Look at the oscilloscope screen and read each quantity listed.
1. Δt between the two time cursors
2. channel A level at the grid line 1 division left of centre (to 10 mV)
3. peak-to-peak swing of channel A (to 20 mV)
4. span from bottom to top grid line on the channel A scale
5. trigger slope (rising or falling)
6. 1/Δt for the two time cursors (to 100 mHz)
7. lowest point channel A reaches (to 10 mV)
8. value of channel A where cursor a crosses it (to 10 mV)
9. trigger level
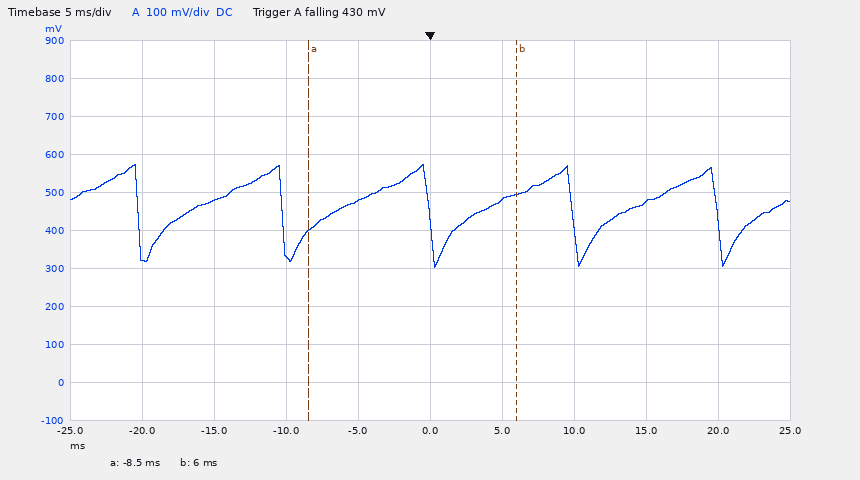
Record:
14.5 ms
480 mV
280 mV
1 V
falling
69.0 Hz
300 mV
400 mV
430 mV
